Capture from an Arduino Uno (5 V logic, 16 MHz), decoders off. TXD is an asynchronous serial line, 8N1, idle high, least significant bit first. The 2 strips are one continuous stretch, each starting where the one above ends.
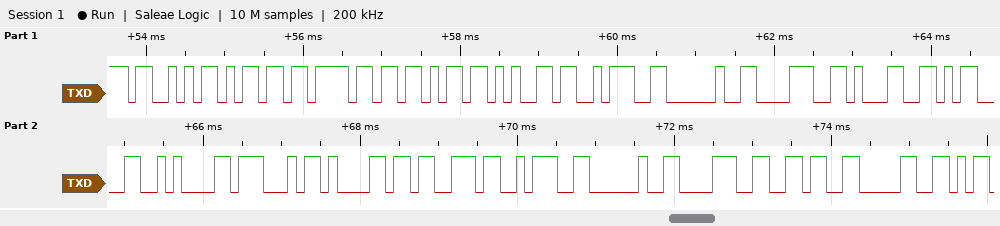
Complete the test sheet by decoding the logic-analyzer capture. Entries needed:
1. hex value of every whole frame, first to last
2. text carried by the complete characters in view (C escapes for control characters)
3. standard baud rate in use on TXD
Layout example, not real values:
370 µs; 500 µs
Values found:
53 6D 6F 6B 65 3A 20 38 31 0D 0A 47 61 73 3A 20 38 36 30; "Smoke: 81\r\nGas: 860"; 9600 baud
